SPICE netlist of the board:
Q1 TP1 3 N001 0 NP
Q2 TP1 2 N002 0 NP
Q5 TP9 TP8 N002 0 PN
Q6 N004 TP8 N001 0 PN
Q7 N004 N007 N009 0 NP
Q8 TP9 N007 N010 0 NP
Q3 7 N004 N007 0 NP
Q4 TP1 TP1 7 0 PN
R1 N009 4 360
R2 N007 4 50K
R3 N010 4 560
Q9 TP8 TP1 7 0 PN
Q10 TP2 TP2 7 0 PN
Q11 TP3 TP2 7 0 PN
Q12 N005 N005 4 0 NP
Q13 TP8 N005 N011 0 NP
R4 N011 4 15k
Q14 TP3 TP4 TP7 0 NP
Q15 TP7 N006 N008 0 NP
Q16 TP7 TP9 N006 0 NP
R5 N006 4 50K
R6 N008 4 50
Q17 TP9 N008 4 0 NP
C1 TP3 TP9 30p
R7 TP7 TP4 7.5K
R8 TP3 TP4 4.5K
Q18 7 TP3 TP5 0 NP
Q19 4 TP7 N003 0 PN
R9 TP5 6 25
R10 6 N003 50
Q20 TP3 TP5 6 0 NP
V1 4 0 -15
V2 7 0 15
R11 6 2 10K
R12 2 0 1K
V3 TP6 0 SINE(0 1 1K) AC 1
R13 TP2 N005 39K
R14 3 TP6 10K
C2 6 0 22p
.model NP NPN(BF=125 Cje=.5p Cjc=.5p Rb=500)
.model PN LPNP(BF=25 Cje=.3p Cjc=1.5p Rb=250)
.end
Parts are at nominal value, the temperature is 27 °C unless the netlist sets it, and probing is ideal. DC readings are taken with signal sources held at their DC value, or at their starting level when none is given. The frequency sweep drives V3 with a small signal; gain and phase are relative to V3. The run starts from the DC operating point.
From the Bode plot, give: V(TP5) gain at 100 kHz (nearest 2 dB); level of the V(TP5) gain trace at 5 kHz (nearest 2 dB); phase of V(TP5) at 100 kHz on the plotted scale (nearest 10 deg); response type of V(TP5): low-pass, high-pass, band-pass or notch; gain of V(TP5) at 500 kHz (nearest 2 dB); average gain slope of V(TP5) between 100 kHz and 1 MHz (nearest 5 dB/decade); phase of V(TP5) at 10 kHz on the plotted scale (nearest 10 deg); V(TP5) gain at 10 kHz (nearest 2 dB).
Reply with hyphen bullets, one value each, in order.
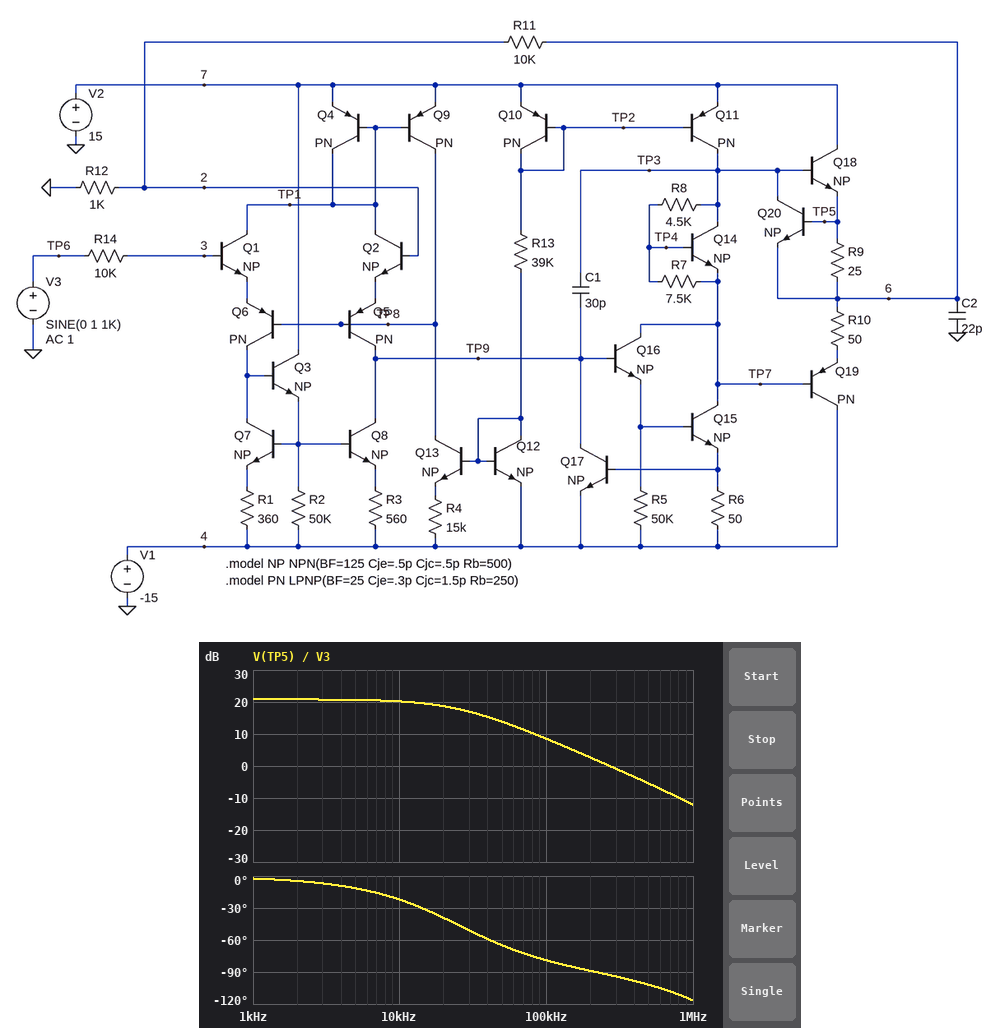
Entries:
- 8 dB
- 20 dB
- -80 deg
- low-pass
- -6 dB
- -20 dB/decade
- -20 deg
- 20 dB
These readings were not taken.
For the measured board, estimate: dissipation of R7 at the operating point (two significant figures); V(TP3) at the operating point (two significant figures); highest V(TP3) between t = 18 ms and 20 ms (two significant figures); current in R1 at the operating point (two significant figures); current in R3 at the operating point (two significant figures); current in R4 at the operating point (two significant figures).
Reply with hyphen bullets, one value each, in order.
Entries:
- 77 µW
- 610 mV
- 12 V
- 3.9 µA
- 3.8 µA
- 8.0 µA
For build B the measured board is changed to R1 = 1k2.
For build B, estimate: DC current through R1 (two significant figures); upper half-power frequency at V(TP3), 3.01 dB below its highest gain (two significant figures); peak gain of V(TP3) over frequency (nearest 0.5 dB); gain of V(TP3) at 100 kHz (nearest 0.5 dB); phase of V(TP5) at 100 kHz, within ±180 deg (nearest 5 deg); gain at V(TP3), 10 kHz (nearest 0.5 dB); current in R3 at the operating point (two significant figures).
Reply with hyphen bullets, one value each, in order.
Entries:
- 3.7 µA
- 30 kHz
- 23.5 dB
- 12.5 dB
- -75 deg
- 23.0 dB
- 4.0 µA
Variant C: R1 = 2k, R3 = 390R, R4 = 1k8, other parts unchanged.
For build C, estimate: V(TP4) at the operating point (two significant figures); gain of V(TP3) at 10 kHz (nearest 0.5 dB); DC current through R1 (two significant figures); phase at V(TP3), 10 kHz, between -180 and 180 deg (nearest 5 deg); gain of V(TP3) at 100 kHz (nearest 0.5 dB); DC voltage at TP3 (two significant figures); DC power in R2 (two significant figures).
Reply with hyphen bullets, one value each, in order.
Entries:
- 590 mV
- 21.5 dB
- 14 µA
- 0 deg
- 21.0 dB
- 1.1 V
- 9.6 µW
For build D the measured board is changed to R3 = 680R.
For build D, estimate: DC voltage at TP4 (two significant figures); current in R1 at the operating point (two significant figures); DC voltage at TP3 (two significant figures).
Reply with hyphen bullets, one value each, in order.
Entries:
- 120 mV
- 4.0 µA
- 590 mV
